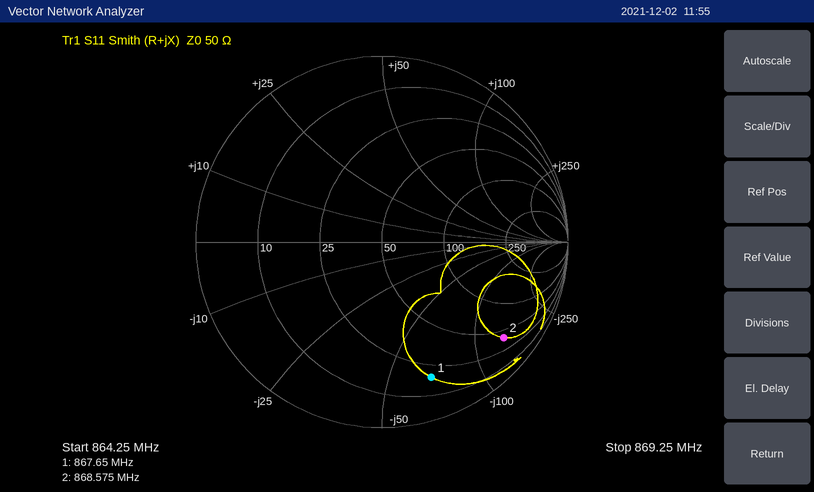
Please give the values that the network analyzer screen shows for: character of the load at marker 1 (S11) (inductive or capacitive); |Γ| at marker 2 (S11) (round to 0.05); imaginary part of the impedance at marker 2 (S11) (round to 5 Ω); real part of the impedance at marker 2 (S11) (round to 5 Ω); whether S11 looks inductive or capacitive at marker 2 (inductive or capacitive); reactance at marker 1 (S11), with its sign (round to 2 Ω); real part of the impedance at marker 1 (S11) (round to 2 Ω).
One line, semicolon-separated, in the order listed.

capacitive; 0.85; -135 Ω; 40 Ω; capacitive; -68 Ω; 18 Ω
